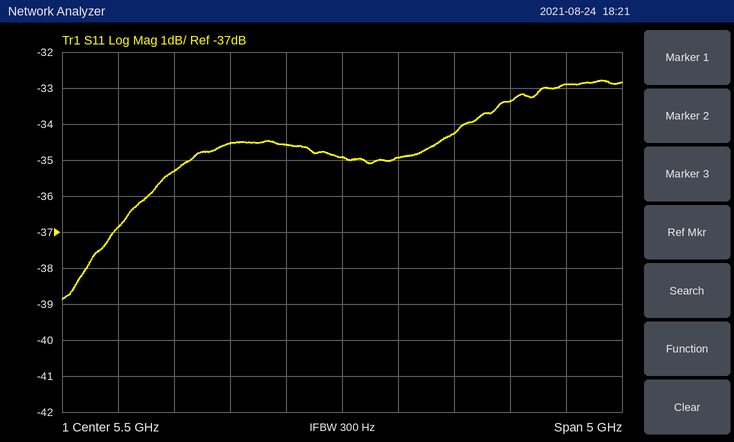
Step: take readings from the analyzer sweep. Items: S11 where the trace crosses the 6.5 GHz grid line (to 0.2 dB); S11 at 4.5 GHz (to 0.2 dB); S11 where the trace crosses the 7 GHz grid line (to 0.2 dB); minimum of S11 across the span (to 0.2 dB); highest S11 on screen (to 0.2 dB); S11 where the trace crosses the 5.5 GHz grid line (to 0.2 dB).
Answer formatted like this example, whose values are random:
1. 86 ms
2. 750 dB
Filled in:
1. -34.2 dB
2. -34.6 dB
3. -33.4 dB
4. -38.8 dB
5. -32.8 dB
6. -35.0 dB
